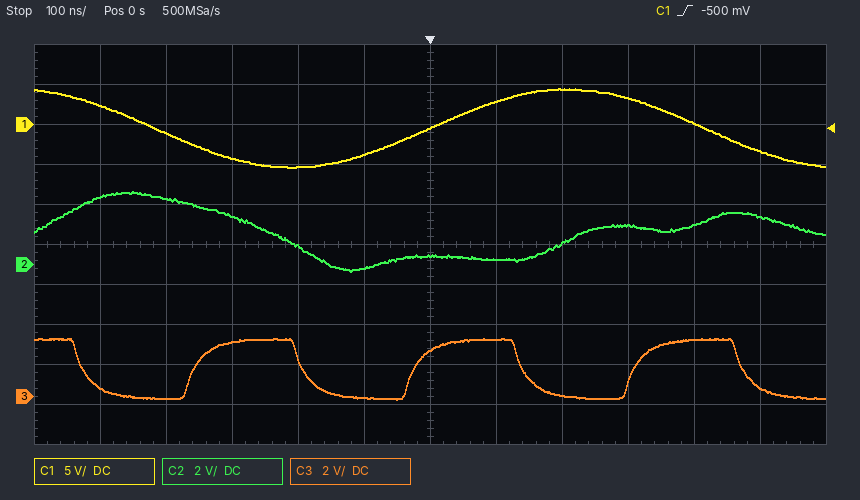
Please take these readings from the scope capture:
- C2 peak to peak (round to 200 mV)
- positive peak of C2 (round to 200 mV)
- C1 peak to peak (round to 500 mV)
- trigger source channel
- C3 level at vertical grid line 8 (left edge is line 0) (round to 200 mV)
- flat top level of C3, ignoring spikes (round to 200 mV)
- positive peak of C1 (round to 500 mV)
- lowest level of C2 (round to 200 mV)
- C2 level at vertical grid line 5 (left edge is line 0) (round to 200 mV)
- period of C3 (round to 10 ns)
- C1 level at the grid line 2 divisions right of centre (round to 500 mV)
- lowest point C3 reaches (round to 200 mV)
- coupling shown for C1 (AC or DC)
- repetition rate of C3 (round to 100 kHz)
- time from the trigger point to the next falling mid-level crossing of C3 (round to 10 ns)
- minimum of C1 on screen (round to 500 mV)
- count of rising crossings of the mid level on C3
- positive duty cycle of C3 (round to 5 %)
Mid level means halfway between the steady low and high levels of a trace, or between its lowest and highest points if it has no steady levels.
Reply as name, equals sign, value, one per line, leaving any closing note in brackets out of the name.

C2 peak to peak = 4.0 V
positive peak of C2 = 3.6 V
C1 peak to peak = 10.0 V
trigger source channel = C1
C3 level at vertical grid line 8 (left edge is line 0) = 0.0 V
flat top level of C3, ignoring spikes = 2.8 V
positive peak of C1 = 4.5 V
lowest level of C2 = -400 mV
C2 level at vertical grid line 5 (left edge is line 0) = -200 mV
period of C3 = 330 ns
C1 level at the grid line 2 divisions right of centre = 4.5 V
lowest point C3 reaches = -200 mV
coupling shown for C1 = DC
repetition rate of C3 = 3.0 MHz
time from the trigger point to the next falling mid-level crossing of C3 = 140 ns
minimum of C1 on screen = -5.5 V
count of rising crossings of the mid level on C3 = 3
positive duty cycle of C3 = 50 %
